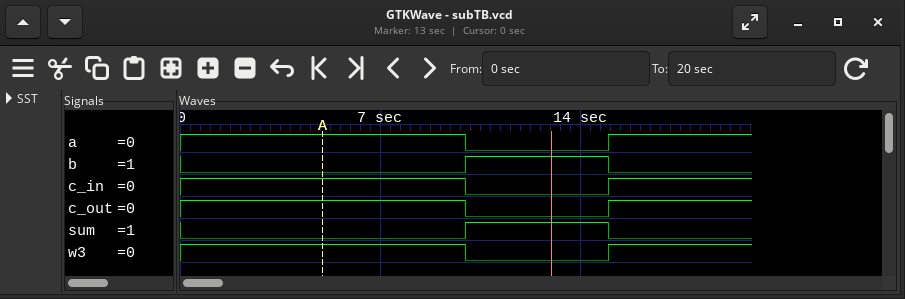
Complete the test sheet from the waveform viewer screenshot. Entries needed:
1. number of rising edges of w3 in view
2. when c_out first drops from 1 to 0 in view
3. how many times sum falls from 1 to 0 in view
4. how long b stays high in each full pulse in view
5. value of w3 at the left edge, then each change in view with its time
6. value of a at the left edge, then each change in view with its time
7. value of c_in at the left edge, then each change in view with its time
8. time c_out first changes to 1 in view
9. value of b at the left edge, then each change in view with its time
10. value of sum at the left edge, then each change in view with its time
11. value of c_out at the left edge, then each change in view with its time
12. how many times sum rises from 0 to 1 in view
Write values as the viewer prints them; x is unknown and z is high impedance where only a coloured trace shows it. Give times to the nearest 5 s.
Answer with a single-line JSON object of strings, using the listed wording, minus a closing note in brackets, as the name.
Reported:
{"number of rising edges of w3 in view": "1", "when c_out first drops from 1 to 0 in view": "10 s", "how many times sum falls from 1 to 0 in view": "1", "how long b stays high in each full pulse in view": "5 s", "value of w3 at the left edge, then each change in view with its time": "1, 0 at 10 s, 1 at 15 s", "value of a at the left edge, then each change in view with its time": "1, 0 at 10 s, 1 at 15 s", "value of c_in at the left edge, then each change in view with its time": "1, 0 at 10 s, 1 at 15 s", "time c_out first changes to 1 in view": "15 s", "value of b at the left edge, then each change in view with its time": "0, 1 at 10 s, 0 at 15 s", "value of sum at the left edge, then each change in view with its time": "0, 1 at 10 s, 0 at 15 s", "value of c_out at the left edge, then each change in view with its time": "1, 0 at 10 s, 1 at 15 s", "how many times sum rises from 0 to 1 in view": "1"}
